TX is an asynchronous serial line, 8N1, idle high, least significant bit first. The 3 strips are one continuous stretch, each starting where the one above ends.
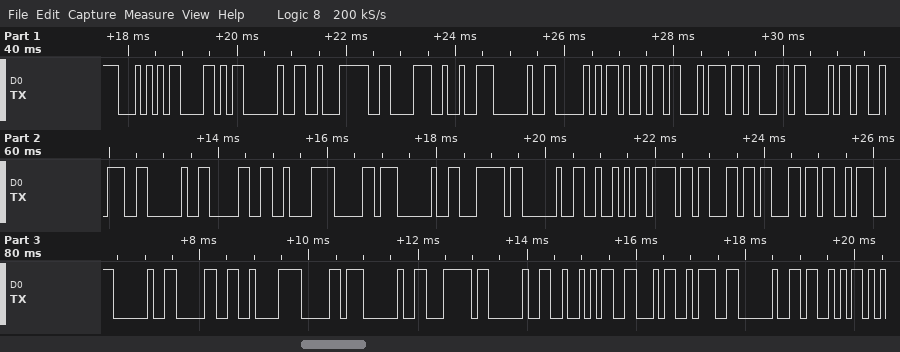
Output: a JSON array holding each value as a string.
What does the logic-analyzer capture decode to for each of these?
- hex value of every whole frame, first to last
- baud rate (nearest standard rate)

["54 58 20 E2 86 92 20 50 69 74 63 68 3A 20 30 C2 B0 20 7C 20 52 6F 6C 6C 3A 20 30 C2 B0 20 7C 20 52 46 3A 20 53", "9600 baud"]
